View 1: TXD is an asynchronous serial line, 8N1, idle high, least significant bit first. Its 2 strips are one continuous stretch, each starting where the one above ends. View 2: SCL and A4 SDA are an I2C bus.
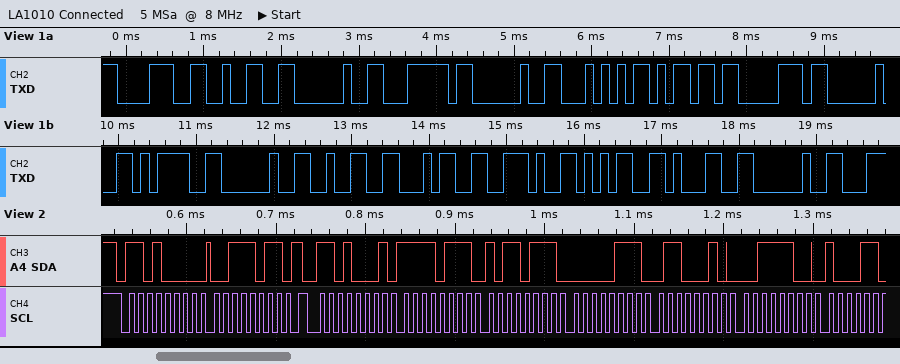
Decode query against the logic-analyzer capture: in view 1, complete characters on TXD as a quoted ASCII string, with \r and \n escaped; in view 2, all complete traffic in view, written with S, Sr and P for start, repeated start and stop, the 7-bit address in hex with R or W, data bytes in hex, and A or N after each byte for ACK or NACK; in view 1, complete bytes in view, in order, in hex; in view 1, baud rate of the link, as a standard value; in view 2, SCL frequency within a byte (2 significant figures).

"82 | Tmp = 24.51 "
S 68W A 3B A Sr 68R A F7 A B7 A 07 A 62 A 3C A
38 32 20 7C 20 54 6D 70 20 3D 20 32 34 2E 35 31 20
9600 baud
100 kHz
